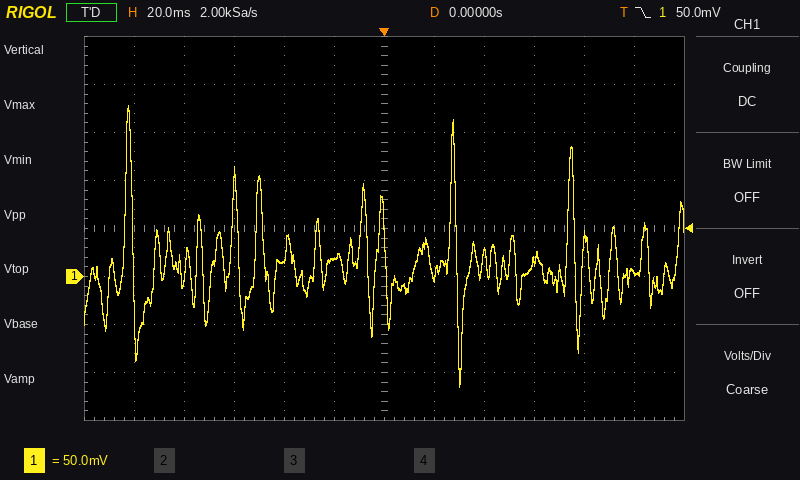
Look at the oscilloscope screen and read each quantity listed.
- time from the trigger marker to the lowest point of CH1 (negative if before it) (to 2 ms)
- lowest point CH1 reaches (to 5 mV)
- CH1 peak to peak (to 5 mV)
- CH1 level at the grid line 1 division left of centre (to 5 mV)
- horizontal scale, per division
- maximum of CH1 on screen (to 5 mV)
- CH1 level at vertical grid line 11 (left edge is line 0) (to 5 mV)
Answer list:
+30 ms
-115 mV
295 mV
20 mV
20 ms
180 mV
5 mV
